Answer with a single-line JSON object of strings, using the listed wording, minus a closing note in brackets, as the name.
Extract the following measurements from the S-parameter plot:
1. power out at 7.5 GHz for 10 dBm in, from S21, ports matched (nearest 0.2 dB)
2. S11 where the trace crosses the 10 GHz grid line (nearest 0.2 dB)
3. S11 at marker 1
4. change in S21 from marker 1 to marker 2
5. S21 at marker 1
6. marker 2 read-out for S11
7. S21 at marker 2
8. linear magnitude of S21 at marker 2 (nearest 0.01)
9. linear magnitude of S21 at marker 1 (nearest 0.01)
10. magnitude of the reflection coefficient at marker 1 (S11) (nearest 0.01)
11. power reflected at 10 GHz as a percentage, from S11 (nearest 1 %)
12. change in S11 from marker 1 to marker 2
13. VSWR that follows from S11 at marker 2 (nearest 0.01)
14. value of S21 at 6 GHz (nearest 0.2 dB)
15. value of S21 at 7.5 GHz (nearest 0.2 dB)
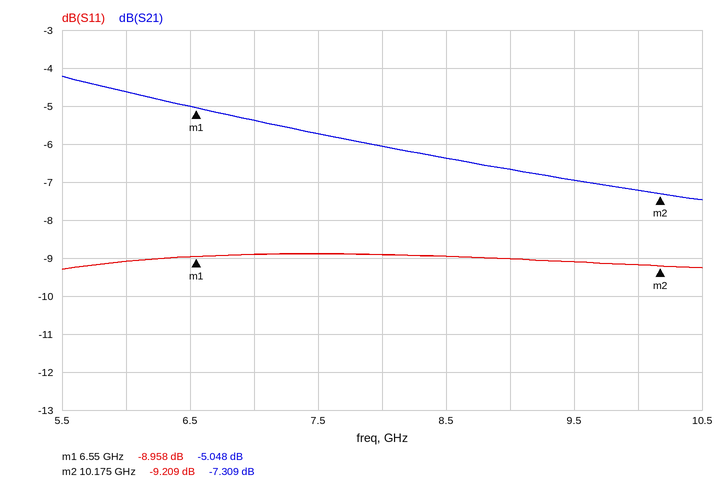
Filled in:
{"power out at 7.5 GHz for 10 dBm in, from S21, ports matched": "4.2 dBm", "S11 where the trace crosses the 10 GHz grid line": "-9.2 dB", "S11 at marker 1": "-8.958 dB", "change in S21 from marker 1 to marker 2": "-2.261 dB", "S21 at marker 1": "-5.048 dB", "marker 2 read-out for S11": "-9.209 dB", "S21 at marker 2": "-7.309 dB", "linear magnitude of S21 at marker 2": "0.43", "linear magnitude of S21 at marker 1": "0.56", "magnitude of the reflection coefficient at marker 1 (S11)": "0.36", "power reflected at 10 GHz as a percentage, from S11": "12 %", "change in S11 from marker 1 to marker 2": "-0.251 dB", "VSWR that follows from S11 at marker 2": "2.06", "value of S21 at 6 GHz": "-4.6 dB", "value of S21 at 7.5 GHz": "-5.8 dB"}
